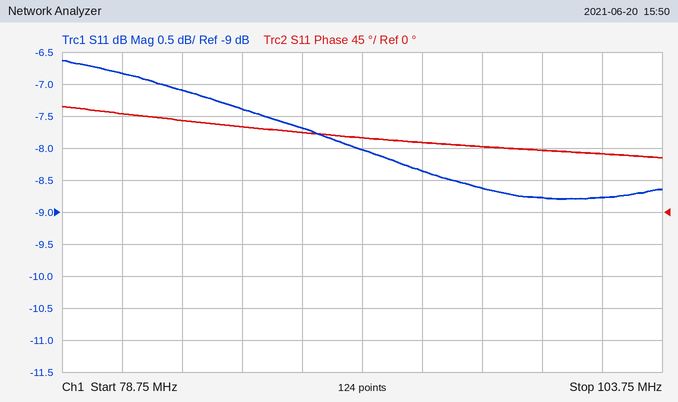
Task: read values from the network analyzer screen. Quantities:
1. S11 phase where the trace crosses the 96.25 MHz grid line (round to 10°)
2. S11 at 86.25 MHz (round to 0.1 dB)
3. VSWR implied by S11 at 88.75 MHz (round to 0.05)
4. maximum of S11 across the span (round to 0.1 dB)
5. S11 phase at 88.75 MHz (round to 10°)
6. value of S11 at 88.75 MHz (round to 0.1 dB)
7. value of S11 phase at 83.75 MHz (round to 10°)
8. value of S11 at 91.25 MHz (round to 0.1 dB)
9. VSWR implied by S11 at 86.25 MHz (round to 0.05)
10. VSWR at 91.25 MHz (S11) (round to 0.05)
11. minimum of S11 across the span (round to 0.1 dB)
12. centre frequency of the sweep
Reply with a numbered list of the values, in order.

1. 90°
2. -7.4 dB
3. 2.40
4. -6.6 dB
5. 110°
6. -7.7 dB
7. 130°
8. -8.0 dB
9. 2.50
10. 2.30
11. -8.8 dB
12. 91.25 MHz
